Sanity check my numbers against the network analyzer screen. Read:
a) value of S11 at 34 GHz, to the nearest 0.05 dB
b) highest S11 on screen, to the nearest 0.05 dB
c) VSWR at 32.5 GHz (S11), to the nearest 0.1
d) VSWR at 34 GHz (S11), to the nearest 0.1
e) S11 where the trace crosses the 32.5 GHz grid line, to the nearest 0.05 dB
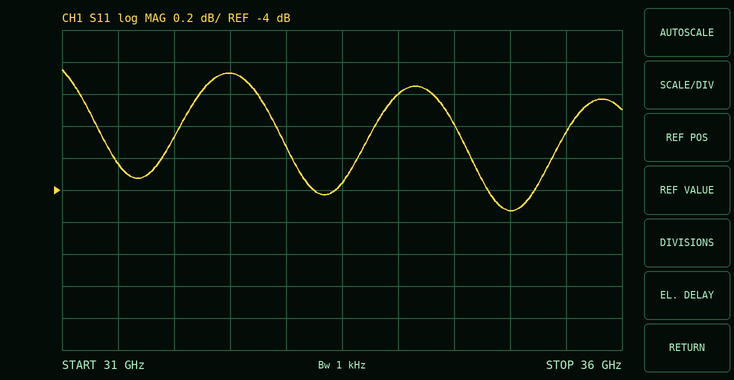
-3.40 dB
-3.25 dB
5.4
5.2
-3.25 dB
